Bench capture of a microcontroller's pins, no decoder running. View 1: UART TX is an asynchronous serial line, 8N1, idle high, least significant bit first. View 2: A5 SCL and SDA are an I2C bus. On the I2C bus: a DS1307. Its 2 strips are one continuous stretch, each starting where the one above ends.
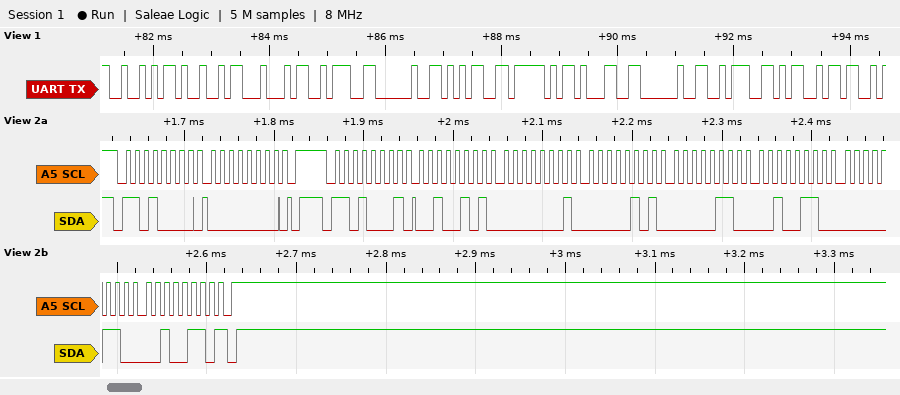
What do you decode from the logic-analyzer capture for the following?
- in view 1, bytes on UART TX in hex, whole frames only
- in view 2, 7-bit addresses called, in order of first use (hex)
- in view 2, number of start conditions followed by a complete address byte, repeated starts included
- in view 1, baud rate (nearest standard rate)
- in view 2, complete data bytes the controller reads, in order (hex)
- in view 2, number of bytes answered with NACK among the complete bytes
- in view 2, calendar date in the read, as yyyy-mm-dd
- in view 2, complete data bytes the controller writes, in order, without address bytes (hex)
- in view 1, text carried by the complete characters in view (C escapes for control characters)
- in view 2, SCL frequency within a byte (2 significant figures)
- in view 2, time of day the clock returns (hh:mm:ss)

52 49 44 3A 20 35 5F 31 20 3A 4D
0x68
2
9600 baud
25 01 05 06 26 06 26
1
2026-06-26
00
"RID: 5_1 :M"
100 kHz
05:01:25
